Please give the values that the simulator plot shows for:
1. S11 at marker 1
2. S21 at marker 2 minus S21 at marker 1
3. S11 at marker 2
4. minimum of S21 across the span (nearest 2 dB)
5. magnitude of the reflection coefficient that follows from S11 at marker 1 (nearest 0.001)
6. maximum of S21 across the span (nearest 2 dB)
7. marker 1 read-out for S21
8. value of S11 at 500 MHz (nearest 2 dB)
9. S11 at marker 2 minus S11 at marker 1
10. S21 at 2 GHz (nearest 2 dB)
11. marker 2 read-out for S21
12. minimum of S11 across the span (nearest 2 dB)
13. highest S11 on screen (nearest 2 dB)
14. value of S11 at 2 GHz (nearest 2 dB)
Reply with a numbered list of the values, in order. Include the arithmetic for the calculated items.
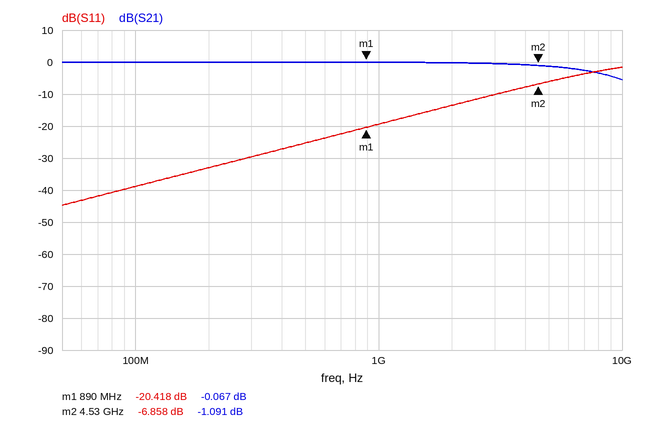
1. -20.418 dB
2. -1.091 − (-0.067) = -1.024 dB
3. -6.858 dB
4. -6 dB
5. 10^(-20.418/20) ≈ 0.095
6. 0 dB
7. -0.067 dB
8. -26 dB
9. -6.858 − (-20.418) = 13.560 dB
10. 0 dB
11. -1.091 dB
12. -44 dB
13. -2 dB
14. -14 dB
